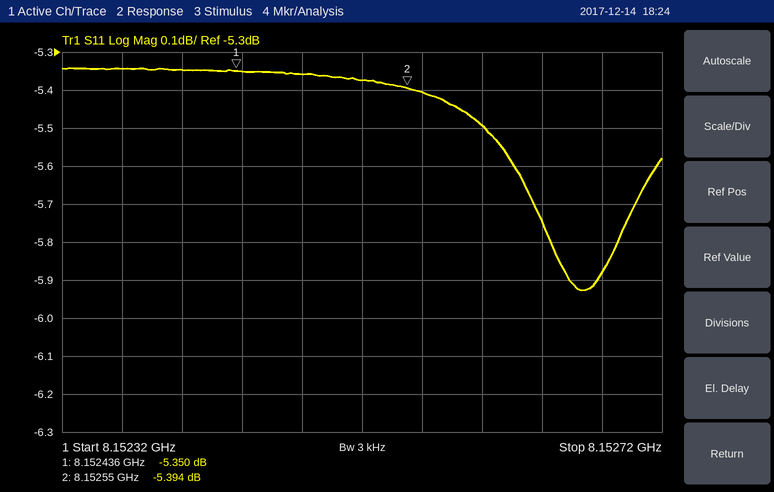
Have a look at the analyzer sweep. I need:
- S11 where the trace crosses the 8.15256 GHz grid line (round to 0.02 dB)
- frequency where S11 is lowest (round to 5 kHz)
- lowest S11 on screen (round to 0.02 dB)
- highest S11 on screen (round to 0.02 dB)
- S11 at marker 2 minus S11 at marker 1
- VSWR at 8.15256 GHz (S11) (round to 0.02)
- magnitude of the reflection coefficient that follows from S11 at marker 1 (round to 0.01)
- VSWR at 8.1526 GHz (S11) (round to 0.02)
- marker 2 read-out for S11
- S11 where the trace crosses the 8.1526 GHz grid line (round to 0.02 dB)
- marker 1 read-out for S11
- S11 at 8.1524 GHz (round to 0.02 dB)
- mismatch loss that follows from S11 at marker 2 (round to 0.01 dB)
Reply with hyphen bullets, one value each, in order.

- -5.40 dB
- 8.152665 GHz
- -5.92 dB
- -5.34 dB
- -0.044 dB
- 3.32
- 0.54
- 3.26
- -5.394 dB
- -5.50 dB
- -5.350 dB
- -5.34 dB
- 1.48 dB
